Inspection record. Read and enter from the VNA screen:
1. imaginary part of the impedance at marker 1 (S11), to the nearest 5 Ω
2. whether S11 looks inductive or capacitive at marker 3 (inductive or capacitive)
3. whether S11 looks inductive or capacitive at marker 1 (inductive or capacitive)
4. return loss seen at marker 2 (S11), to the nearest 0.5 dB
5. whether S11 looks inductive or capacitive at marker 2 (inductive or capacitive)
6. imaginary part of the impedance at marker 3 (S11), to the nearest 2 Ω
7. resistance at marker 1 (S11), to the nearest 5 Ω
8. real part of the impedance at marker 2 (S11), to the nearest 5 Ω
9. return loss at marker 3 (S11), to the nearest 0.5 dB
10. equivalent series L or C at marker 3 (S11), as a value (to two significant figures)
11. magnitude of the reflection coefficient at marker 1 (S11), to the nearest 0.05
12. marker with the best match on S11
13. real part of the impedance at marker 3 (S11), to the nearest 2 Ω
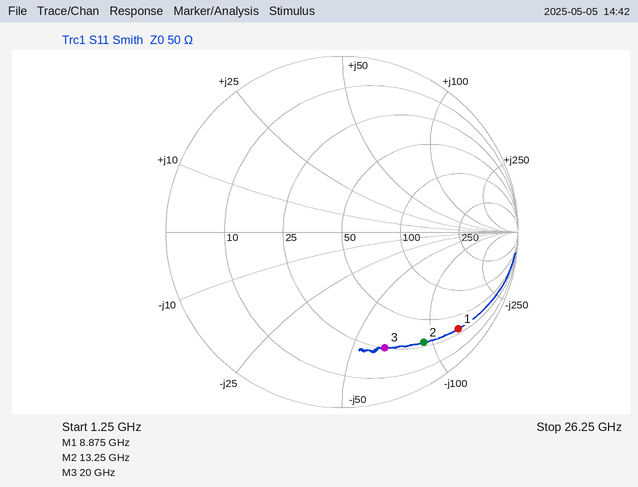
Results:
-130 Ω
capacitive
capacitive
2.0 dB
capacitive
-66 Ω
30 Ω
30 Ω
3.0 dB
120 fF
0.85
marker 3
26 Ω
